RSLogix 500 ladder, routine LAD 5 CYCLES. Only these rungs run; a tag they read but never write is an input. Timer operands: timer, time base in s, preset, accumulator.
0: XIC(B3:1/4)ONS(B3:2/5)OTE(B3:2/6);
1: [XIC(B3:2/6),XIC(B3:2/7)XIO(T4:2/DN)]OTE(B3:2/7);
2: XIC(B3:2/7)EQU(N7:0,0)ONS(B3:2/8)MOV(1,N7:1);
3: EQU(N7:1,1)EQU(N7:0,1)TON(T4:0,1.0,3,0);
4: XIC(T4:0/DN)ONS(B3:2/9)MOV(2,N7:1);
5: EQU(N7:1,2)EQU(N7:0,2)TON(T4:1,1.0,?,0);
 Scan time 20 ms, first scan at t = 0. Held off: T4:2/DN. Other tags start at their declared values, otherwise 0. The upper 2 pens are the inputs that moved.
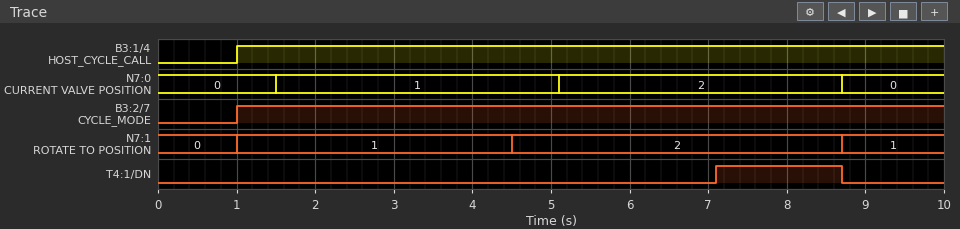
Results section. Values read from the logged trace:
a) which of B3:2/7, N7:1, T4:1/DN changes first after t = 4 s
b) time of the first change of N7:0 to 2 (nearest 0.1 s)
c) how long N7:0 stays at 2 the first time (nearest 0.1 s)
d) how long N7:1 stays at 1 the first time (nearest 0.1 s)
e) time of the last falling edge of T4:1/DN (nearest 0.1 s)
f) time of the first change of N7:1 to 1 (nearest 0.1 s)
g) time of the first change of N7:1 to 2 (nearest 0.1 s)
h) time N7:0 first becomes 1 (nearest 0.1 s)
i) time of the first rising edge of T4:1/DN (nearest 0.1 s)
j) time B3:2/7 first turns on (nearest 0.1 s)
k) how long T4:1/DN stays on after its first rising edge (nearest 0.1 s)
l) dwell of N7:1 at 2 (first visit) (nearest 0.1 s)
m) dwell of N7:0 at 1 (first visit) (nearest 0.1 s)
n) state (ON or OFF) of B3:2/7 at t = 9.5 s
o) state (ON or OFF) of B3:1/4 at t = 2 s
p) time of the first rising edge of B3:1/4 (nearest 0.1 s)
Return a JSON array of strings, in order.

["N7:1", "5.1 s", "3.6 s", "3.5 s", "8.7 s", "1.0 s", "4.5 s", "1.5 s", "7.1 s", "1.0 s", "1.6 s", "4.2 s", "3.6 s", "ON", "ON", "1.0 s"]
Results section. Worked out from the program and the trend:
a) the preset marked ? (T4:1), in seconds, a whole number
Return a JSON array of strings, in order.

["2 s"]
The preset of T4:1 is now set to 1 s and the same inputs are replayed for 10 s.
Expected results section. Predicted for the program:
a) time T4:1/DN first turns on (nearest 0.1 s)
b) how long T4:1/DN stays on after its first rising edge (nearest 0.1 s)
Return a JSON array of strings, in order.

["6.1 s", "2.6 s"]
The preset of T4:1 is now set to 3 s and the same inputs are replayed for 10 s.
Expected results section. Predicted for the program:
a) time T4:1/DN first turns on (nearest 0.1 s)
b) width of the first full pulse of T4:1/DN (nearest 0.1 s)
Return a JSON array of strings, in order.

["8.1 s", "0.6 s"]
